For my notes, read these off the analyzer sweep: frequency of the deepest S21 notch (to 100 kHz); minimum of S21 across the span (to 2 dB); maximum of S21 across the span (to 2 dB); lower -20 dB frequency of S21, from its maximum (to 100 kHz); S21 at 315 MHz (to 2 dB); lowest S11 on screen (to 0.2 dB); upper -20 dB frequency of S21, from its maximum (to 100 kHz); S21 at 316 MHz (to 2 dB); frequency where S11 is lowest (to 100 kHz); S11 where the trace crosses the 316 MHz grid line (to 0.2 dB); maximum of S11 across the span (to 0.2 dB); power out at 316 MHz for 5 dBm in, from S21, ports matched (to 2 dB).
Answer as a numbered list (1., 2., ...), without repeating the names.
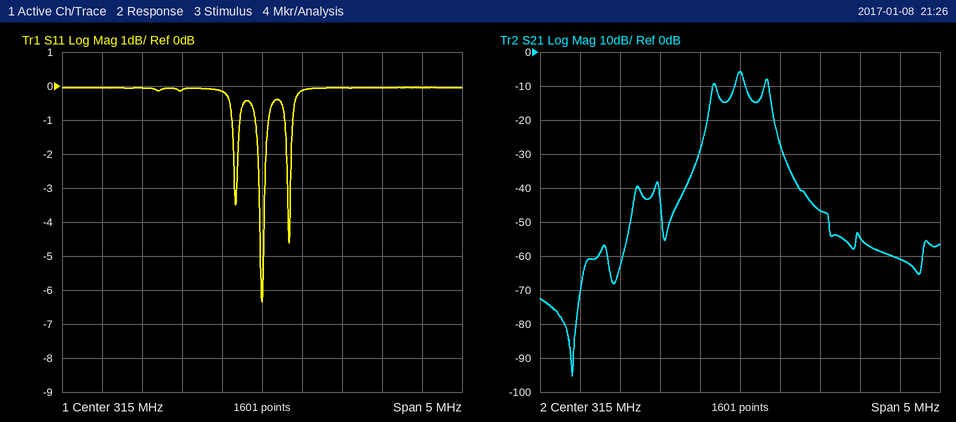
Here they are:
1. 312.9 MHz
2. -96 dB
3. -6 dB
4. 314.5 MHz
5. -6 dB
6. -6.4 dB
7. 315.5 MHz
8. -46 dB
9. 315.0 MHz
10. 0.0 dB
11. 0.0 dB
12. -42 dBm
